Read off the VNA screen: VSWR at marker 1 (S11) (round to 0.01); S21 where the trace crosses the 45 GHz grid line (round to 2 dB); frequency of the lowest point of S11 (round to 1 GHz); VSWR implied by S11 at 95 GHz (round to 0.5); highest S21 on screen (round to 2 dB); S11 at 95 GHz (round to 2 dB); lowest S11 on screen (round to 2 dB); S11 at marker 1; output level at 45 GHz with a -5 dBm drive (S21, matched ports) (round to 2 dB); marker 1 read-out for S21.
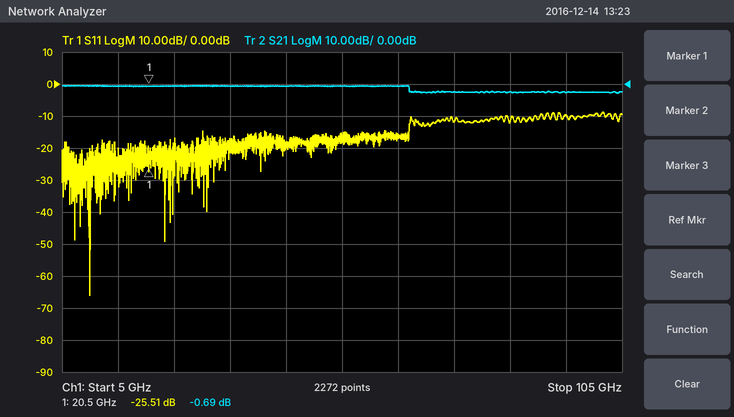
1.11
0 dB
10 GHz
2.0
0 dB
-10 dB
-66 dB
-25.51 dB
-6 dBm
-0.69 dB
